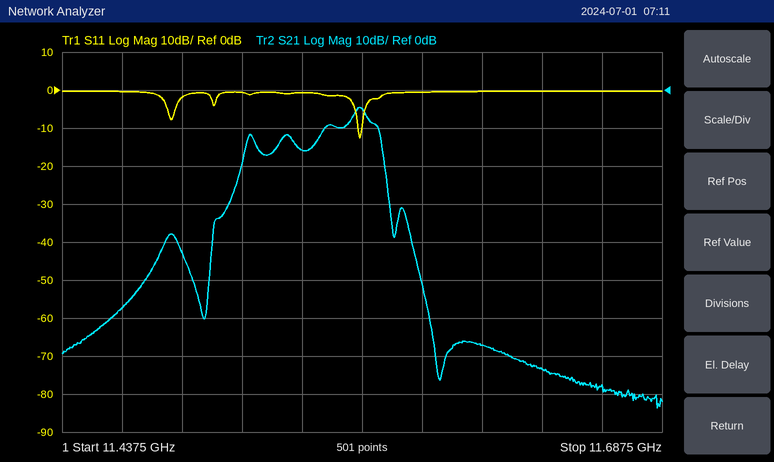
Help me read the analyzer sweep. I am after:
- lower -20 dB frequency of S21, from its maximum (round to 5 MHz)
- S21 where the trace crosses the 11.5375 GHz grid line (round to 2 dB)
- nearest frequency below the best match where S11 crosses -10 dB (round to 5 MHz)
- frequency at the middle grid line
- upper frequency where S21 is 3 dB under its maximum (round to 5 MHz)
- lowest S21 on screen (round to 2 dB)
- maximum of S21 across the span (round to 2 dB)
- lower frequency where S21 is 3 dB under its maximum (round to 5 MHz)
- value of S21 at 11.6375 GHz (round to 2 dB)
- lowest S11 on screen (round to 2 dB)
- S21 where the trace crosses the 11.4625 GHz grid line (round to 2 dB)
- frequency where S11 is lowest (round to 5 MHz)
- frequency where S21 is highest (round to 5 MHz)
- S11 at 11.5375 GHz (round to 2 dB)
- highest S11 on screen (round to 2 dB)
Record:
11.510 GHz
-16 dB
11.560 GHz
11.5625 GHz
11.565 GHz
-84 dB
-4 dB
11.560 GHz
-74 dB
-12 dB
-58 dB
11.560 GHz
11.560 GHz
0 dB
0 dB
